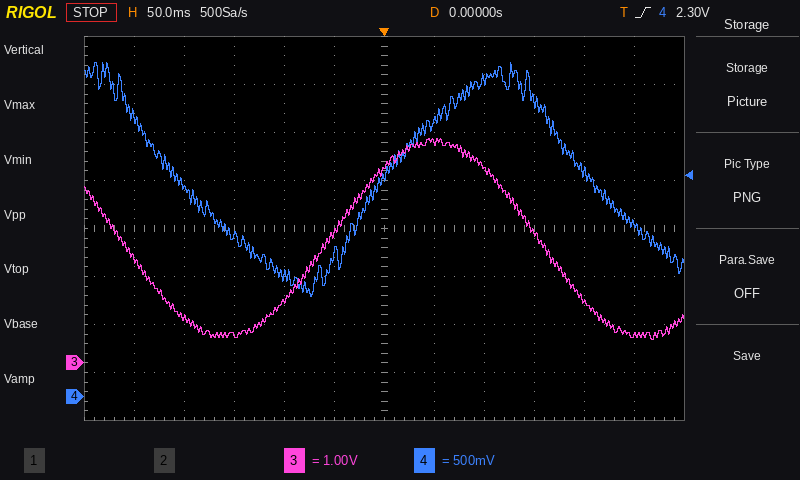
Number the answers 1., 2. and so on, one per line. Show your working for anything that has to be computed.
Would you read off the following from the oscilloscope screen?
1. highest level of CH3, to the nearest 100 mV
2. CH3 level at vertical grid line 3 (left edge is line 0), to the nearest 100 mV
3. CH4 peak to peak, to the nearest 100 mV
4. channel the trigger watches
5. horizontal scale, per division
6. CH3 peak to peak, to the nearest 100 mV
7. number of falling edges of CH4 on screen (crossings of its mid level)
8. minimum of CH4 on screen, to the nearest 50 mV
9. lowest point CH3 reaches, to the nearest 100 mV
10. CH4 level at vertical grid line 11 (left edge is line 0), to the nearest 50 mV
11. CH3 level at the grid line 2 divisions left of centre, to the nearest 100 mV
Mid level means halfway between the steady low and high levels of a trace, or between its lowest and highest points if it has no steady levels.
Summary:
1. 4.7 V
2. 600 mV
3. 2.40 V
4. CH4
5. 50 ms
6. 4.7 V − (500 mV) = 4.2 V
7. 2
8. 1.05 V
9. 500 mV
10. 1.80 V
11. 1.3 V
